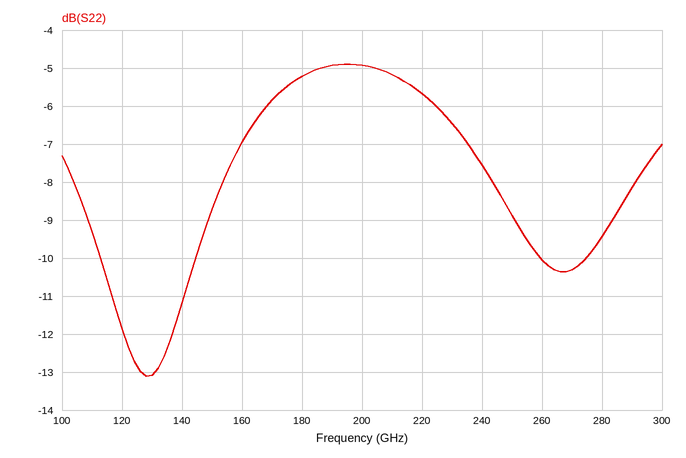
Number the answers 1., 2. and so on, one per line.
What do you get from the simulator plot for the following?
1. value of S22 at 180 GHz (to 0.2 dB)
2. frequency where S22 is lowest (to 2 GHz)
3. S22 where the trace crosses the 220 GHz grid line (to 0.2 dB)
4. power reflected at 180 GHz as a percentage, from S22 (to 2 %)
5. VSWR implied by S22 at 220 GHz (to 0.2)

1. -5.2 dB
2. 128 GHz
3. -5.6 dB
4. 30 %
5. 3.2
